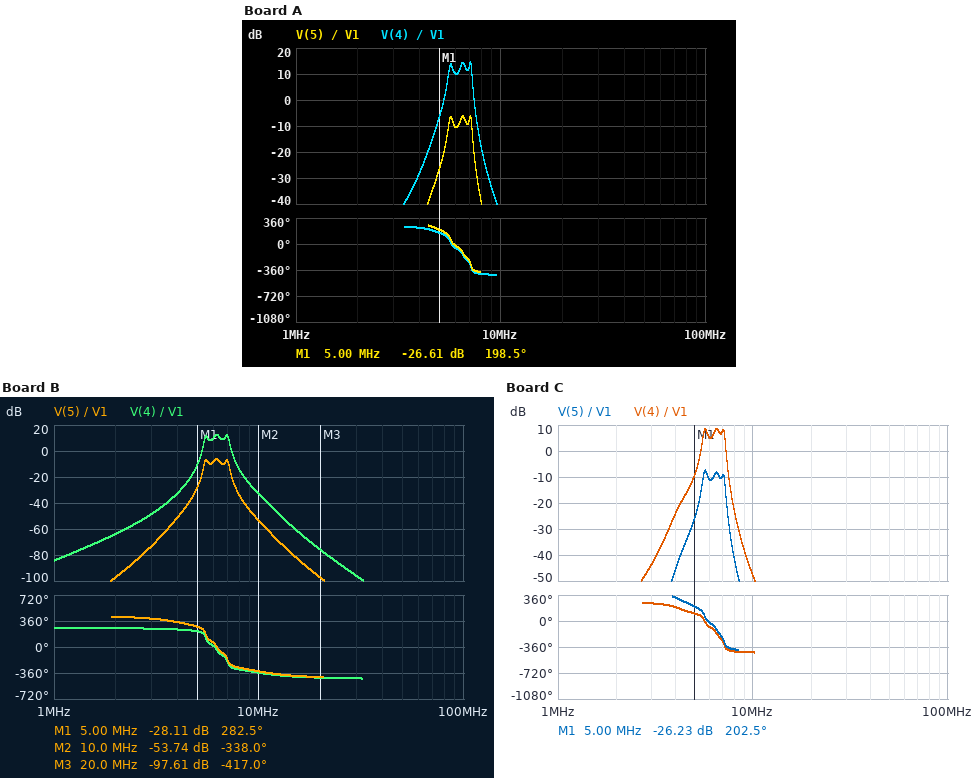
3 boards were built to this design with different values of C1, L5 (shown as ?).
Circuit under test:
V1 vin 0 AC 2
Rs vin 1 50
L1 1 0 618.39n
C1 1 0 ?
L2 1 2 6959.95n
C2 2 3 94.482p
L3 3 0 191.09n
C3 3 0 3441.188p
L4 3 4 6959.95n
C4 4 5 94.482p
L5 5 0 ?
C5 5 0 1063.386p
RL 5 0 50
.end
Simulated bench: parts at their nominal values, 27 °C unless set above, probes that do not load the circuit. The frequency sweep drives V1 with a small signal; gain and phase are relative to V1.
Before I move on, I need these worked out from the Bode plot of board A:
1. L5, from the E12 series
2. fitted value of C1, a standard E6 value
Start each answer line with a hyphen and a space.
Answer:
- 2.2 µH
- 1.5 nF
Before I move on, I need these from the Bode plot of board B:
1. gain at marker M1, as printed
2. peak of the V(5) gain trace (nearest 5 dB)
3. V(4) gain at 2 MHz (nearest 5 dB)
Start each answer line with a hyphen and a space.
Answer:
- -28.11 dB
- -5 dB
- -65 dB
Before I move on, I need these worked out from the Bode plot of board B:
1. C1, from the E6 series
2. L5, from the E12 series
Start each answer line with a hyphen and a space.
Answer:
- 470 pF
- 1.2 µH
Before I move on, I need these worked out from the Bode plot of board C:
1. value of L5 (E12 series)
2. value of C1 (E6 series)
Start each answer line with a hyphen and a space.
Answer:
- 820 nH
- 2.2 nF
